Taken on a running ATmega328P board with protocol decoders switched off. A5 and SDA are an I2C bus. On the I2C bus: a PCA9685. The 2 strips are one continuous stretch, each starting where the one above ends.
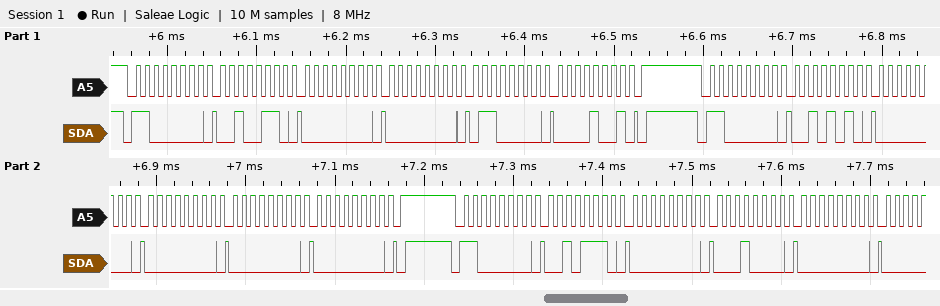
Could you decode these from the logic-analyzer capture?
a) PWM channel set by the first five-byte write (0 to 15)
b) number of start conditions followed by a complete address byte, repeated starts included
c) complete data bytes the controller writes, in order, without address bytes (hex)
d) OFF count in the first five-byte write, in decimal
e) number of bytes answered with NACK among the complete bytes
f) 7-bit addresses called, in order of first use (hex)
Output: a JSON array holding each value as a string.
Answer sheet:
["8", "3", "26 00 00 60 09 2A 00 00 00 00 2E 00 10 00", "2400", "0", "0x60"]
